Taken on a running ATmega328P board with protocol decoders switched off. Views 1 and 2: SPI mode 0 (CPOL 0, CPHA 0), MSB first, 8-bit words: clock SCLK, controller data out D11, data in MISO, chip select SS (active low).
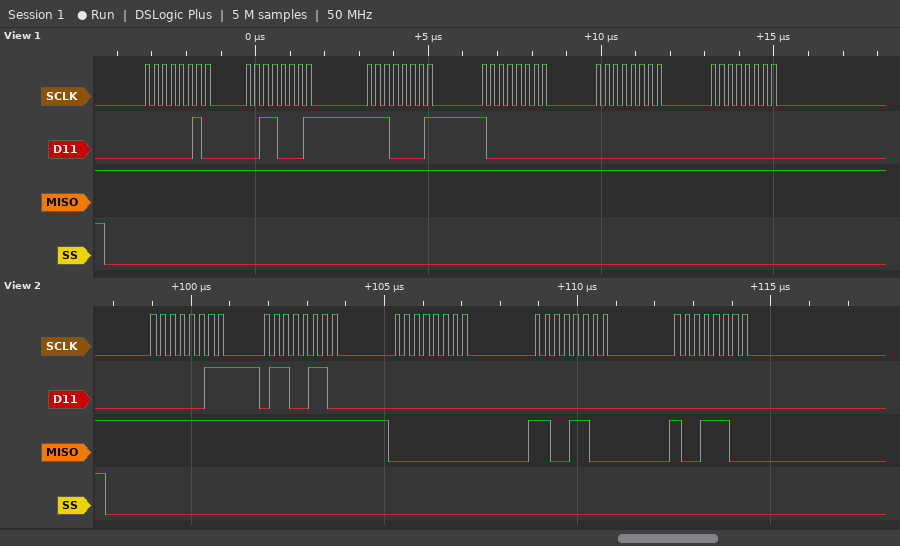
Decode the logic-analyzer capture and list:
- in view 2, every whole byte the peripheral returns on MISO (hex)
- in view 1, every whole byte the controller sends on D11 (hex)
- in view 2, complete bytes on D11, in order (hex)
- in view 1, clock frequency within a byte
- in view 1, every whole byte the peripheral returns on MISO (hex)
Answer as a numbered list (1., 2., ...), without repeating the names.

1. 0xFF 0xFF 0x00 0xCC 0x9C
2. 0x02 0x31 0xE1 0x80 0x00 0x00
3. 0x03 0x66 0x00 0x00 0x00
4. 4 MHz
5. 0xFF 0xFF 0xFF 0xFF 0xFF 0xFF
